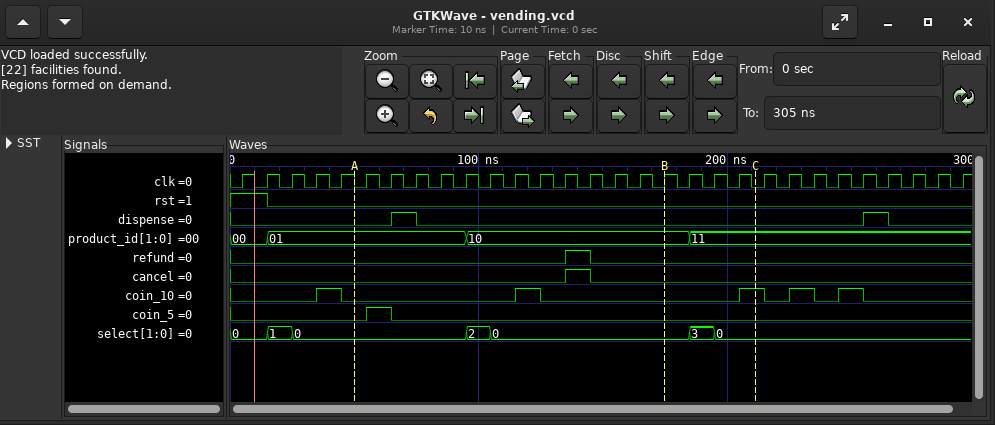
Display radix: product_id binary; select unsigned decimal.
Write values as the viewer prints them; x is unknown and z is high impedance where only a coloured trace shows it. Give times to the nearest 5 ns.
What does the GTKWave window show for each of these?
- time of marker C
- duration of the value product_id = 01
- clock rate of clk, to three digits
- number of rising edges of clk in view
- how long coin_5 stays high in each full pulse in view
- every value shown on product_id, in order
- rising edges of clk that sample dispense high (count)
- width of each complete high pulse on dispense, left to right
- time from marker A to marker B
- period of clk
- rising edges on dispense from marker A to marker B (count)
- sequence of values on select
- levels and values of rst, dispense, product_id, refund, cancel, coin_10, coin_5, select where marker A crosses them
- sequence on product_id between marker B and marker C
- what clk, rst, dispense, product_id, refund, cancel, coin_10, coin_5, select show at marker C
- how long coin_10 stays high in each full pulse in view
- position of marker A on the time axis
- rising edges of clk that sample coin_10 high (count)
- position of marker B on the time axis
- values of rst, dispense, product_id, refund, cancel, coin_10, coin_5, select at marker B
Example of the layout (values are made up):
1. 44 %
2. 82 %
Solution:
1. 210 ns
2. 80 ns
3. 100 MHz
4. 30
5. 10 ns
6. 00, 01, 10, 11
7. 2
8. 10 ns, 10 ns
9. 125 ns
10. 10 ns
11. 1
12. 0, 1, 0, 2, 0, 3, 0
13. rst=0, dispense=0, product_id=01, refund=0, cancel=0, coin_10=0, coin_5=0, select=0
14. 10, 11
15. clk=0, rst=0, dispense=0, product_id=11, refund=0, cancel=0, coin_10=1, coin_5=0, select=0
16. 10 ns, 10 ns, 10 ns, 10 ns, 10 ns
17. 50 ns
18. 5
19. 175 ns
20. rst=0, dispense=0, product_id=10, refund=0, cancel=0, coin_10=0, coin_5=0, select=0
